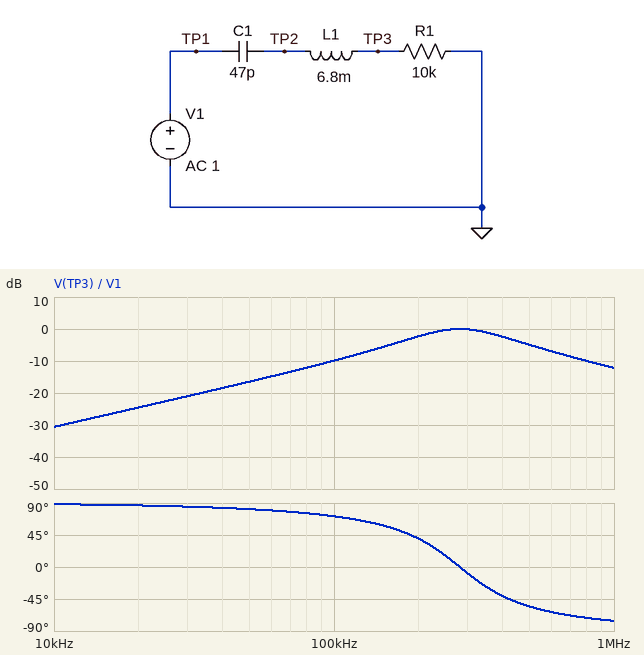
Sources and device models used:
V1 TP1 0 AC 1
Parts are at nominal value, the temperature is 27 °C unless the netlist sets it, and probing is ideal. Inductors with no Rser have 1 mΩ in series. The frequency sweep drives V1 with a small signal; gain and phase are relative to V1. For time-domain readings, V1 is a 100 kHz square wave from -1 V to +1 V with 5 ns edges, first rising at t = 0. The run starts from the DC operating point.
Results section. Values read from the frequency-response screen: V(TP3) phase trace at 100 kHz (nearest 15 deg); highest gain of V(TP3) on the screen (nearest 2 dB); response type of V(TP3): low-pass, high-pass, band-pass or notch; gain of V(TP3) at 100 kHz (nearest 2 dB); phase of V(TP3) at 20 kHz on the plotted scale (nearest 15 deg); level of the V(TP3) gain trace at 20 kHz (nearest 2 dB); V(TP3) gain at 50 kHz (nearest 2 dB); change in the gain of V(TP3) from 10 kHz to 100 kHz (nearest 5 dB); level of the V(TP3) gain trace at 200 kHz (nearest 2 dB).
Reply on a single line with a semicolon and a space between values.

75 deg; 0 dB; band-pass; -10 dB; 90 deg; -24 dB; -16 dB; 20 dB; -2 dB
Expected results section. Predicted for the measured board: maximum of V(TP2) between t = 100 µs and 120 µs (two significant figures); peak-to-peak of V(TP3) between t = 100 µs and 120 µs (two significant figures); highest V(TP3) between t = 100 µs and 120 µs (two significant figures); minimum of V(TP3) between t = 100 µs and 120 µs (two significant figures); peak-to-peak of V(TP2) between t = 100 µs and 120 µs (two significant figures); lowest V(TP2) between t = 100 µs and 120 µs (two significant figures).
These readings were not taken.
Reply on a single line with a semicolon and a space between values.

2.0 V; 2.0 V; 980 mV; -980 mV; 4.0 V; -2.0 V
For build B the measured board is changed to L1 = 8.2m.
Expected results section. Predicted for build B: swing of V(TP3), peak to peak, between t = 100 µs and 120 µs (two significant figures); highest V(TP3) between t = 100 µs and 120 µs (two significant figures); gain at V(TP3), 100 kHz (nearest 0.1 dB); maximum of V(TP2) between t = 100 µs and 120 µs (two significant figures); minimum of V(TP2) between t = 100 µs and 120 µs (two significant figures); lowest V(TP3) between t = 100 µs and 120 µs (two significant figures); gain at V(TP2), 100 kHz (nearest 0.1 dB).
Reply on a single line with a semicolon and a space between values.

1.8 V; 900 mV; -9.7 dB; 1.9 V; -1.9 V; -900 mV; -8.6 dB
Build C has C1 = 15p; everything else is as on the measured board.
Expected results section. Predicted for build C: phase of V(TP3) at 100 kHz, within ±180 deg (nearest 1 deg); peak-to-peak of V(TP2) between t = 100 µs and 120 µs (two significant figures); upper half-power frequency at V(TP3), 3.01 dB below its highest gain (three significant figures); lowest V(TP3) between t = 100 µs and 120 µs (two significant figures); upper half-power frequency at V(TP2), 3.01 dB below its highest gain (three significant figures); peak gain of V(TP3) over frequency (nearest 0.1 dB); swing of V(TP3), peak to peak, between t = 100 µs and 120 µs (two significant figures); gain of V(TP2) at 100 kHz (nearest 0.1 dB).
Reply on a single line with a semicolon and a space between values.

84 deg; 4.1 V; 629 kHz; -690 mV; 726 kHz; 0 dB; 1.4 V; -19.5 dB
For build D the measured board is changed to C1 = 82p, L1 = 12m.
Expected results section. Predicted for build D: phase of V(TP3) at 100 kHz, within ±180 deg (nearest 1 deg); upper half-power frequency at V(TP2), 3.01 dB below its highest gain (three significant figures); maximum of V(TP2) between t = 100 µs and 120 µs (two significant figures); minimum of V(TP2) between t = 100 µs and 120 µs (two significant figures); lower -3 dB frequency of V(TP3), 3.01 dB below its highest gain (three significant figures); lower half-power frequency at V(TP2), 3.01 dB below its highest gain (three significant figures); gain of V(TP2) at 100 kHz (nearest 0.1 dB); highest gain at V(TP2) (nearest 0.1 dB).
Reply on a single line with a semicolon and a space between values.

50 deg; 425 kHz; 2.1 V; -2.1 V; 107 kHz; 123 kHz; -1.9 dB; 4.2 dB
